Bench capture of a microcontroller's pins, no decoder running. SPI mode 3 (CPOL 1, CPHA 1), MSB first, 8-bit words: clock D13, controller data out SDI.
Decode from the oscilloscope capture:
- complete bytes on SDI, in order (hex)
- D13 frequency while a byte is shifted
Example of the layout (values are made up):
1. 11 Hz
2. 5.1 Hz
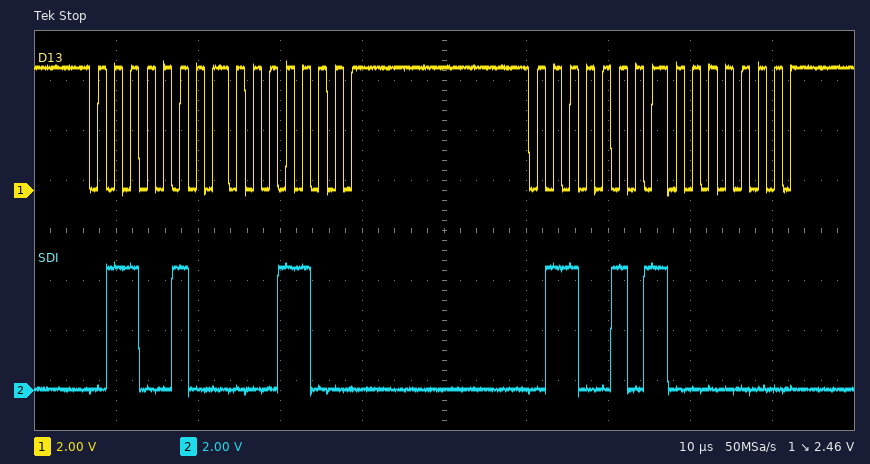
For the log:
1. 0x64 0x18 0x65 0x00
2. 500 kHz
